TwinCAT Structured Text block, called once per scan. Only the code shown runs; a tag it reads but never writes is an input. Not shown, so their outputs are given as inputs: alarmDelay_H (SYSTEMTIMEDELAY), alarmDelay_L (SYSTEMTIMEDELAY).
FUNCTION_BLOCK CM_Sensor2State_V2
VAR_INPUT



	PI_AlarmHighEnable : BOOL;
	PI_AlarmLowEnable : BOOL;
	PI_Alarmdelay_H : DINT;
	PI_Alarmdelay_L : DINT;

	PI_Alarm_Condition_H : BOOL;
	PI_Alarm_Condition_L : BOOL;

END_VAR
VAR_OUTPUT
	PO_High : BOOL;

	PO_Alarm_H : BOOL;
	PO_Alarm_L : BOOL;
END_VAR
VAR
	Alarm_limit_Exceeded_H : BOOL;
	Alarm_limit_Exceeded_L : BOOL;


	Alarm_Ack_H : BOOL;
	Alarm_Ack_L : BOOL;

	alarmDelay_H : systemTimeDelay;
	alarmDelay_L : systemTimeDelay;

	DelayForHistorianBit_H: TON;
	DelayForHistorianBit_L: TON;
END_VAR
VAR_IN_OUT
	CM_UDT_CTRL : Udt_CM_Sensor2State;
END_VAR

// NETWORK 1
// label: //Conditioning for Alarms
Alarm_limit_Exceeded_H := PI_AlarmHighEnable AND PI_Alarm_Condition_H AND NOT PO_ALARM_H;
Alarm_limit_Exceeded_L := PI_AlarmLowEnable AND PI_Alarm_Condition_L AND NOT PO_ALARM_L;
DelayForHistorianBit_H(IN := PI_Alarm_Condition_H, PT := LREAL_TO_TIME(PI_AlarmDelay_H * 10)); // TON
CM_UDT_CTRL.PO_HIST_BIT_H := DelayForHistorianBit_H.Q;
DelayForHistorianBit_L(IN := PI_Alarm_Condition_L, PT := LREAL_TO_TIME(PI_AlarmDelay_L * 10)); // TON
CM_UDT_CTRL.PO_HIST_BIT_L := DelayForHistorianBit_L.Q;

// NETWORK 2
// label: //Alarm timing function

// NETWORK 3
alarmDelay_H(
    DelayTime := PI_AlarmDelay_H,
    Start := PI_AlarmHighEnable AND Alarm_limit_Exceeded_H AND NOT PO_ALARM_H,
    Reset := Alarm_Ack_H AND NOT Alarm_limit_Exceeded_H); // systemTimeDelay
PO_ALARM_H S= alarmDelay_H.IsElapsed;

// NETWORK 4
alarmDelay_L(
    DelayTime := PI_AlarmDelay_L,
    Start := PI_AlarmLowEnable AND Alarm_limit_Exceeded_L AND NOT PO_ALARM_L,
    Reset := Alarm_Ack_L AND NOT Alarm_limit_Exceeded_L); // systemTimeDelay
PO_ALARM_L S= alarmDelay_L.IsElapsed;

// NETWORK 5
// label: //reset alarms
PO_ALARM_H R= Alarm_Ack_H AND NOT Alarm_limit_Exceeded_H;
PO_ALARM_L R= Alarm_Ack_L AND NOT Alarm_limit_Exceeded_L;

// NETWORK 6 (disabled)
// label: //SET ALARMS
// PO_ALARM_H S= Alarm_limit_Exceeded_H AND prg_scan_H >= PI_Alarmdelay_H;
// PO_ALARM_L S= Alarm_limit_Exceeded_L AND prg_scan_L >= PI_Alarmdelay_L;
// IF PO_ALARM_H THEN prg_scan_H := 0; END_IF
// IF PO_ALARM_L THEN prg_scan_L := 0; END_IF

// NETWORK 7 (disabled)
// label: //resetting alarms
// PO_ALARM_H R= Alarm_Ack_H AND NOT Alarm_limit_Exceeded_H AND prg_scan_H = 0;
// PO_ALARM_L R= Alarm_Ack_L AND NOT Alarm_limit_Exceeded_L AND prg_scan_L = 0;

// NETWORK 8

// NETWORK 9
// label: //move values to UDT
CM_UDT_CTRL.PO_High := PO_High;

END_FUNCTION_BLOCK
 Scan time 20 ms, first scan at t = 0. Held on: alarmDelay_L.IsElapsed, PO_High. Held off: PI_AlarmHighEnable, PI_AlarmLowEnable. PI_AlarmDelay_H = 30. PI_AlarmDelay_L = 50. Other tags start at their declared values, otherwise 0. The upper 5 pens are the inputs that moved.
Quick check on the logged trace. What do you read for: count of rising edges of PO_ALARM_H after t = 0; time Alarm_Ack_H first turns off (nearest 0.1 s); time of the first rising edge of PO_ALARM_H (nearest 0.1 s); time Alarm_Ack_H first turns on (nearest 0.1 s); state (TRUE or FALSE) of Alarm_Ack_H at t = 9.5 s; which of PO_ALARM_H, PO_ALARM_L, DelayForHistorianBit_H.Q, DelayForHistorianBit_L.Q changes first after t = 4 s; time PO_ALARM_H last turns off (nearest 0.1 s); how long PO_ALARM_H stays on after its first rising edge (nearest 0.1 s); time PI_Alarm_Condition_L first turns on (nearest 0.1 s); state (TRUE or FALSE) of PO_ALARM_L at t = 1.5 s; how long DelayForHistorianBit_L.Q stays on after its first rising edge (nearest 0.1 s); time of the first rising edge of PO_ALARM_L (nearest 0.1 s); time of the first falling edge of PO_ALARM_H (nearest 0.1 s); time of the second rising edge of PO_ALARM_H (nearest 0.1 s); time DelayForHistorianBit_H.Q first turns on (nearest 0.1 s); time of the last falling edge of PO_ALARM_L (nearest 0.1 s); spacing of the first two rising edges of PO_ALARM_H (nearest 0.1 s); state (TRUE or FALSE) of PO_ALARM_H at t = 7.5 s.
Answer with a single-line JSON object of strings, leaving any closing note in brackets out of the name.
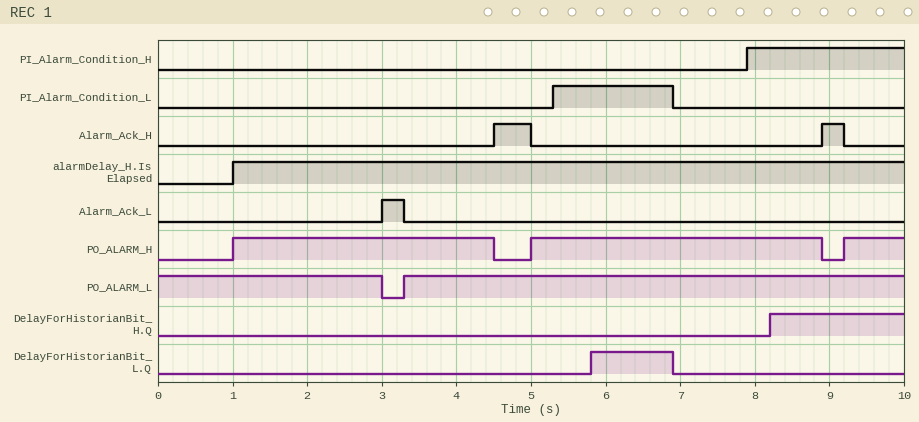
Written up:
{"count of rising edges of PO_ALARM_H after t = 0": "3", "time Alarm_Ack_H first turns off": "5.0 s", "time of the first rising edge of PO_ALARM_H": "1.0 s", "time Alarm_Ack_H first turns on": "4.5 s", "state (TRUE or FALSE) of Alarm_Ack_H at t = 9.5 s": "FALSE", "which of PO_ALARM_H, PO_ALARM_L, DelayForHistorianBit_H.Q, DelayForHistorianBit_L.Q changes first after t = 4 s": "PO_ALARM_H", "time PO_ALARM_H last turns off": "8.9 s", "how long PO_ALARM_H stays on after its first rising edge": "3.5 s", "time PI_Alarm_Condition_L first turns on": "5.3 s", "state (TRUE or FALSE) of PO_ALARM_L at t = 1.5 s": "TRUE", "how long DelayForHistorianBit_L.Q stays on after its first rising edge": "1.1 s", "time of the first rising edge of PO_ALARM_L": "3.3 s", "time of the first falling edge of PO_ALARM_H": "4.5 s", "time of the second rising edge of PO_ALARM_H": "5.0 s", "time DelayForHistorianBit_H.Q first turns on": "8.2 s", "time of the last falling edge of PO_ALARM_L": "3.0 s", "spacing of the first two rising edges of PO_ALARM_H": "4.0 s", "state (TRUE or FALSE) of PO_ALARM_H at t = 7.5 s": "TRUE"}
